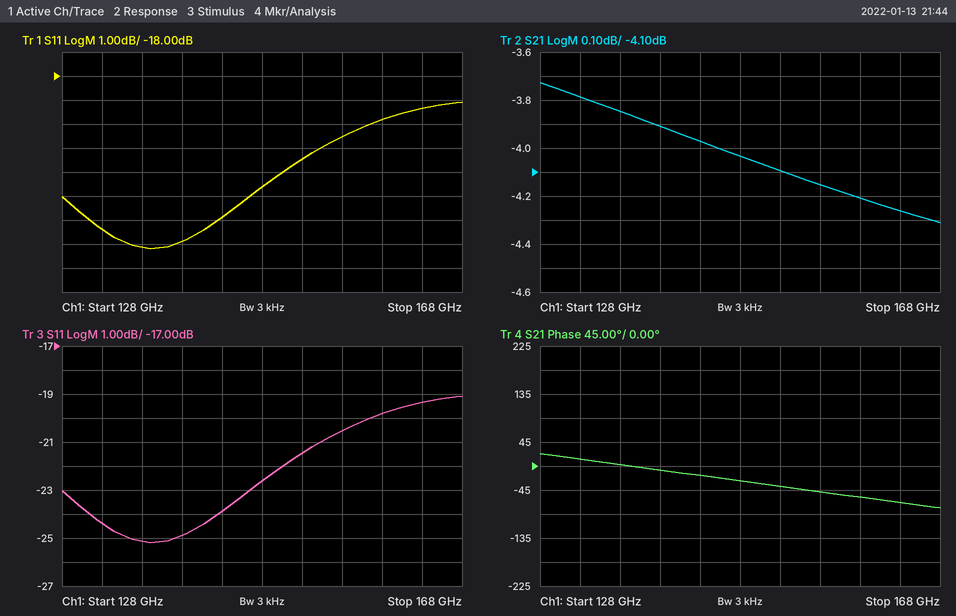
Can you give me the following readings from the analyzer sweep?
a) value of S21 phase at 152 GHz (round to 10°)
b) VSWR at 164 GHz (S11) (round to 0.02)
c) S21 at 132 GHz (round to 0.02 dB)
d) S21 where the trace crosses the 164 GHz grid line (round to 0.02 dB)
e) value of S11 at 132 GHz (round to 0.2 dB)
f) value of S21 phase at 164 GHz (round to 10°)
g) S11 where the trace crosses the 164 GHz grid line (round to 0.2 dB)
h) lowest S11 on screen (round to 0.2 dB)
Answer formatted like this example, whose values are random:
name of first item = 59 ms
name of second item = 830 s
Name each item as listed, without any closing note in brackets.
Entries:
value of S21 phase at 152 GHz = -40°
VSWR at 164 GHz (S11) = 1.24
S21 at 132 GHz = -3.78 dB
S21 where the trace crosses the 164 GHz grid line = -4.26 dB
value of S11 at 132 GHz = -24.4 dB
value of S21 phase at 164 GHz = -70°
S11 where the trace crosses the 164 GHz grid line = -19.4 dB
lowest S11 on screen = -25.2 dB
